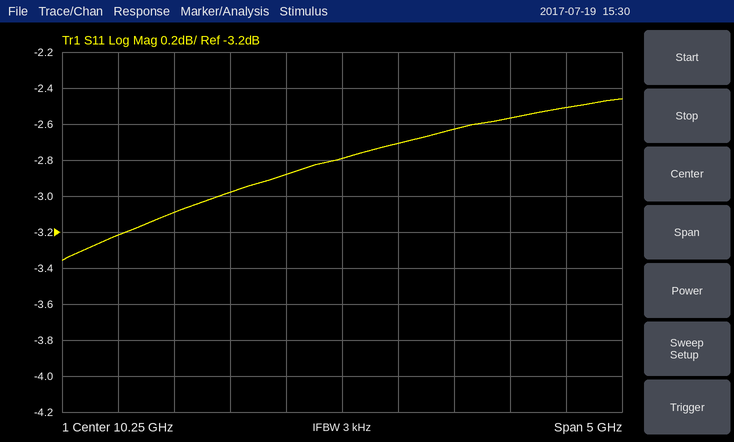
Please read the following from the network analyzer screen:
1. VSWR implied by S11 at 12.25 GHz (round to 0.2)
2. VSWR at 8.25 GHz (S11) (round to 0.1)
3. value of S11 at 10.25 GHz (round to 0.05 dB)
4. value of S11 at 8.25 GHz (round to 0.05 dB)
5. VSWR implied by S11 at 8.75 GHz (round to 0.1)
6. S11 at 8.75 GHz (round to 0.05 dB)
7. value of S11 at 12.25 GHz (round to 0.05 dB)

7.0
5.5
-2.80 dB
-3.20 dB
5.7
-3.10 dB
-2.50 dB
